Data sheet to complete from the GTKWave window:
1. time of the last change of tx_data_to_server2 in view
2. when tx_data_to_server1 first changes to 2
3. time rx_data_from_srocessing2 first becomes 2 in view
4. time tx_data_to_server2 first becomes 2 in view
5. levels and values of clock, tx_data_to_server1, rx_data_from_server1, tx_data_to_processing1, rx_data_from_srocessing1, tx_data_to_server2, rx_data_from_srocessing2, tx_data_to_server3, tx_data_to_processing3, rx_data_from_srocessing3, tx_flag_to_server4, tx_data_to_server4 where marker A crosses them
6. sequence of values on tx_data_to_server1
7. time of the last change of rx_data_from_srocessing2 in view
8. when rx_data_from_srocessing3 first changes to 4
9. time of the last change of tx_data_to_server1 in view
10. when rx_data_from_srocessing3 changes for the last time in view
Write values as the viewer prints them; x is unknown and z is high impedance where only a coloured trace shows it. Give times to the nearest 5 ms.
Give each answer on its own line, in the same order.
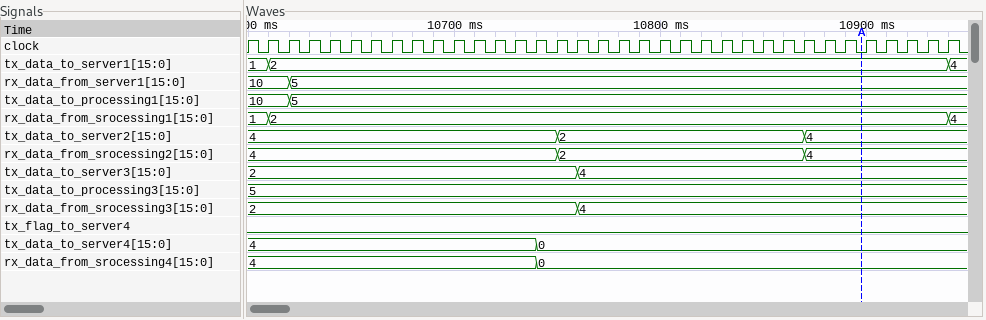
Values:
10870 ms
10610 ms
10750 ms
10750 ms
clock=0, tx_data_to_server1=2, rx_data_from_server1=5, tx_data_to_processing1=5, rx_data_from_srocessing1=2, tx_data_to_server2=4, rx_data_from_srocessing2=4, tx_data_to_server3=4, tx_data_to_processing3=5, rx_data_from_srocessing3=4, tx_flag_to_server4=0, tx_data_to_server4=0
1, 2, 4
10870 ms
10760 ms
10940 ms
10760 ms
